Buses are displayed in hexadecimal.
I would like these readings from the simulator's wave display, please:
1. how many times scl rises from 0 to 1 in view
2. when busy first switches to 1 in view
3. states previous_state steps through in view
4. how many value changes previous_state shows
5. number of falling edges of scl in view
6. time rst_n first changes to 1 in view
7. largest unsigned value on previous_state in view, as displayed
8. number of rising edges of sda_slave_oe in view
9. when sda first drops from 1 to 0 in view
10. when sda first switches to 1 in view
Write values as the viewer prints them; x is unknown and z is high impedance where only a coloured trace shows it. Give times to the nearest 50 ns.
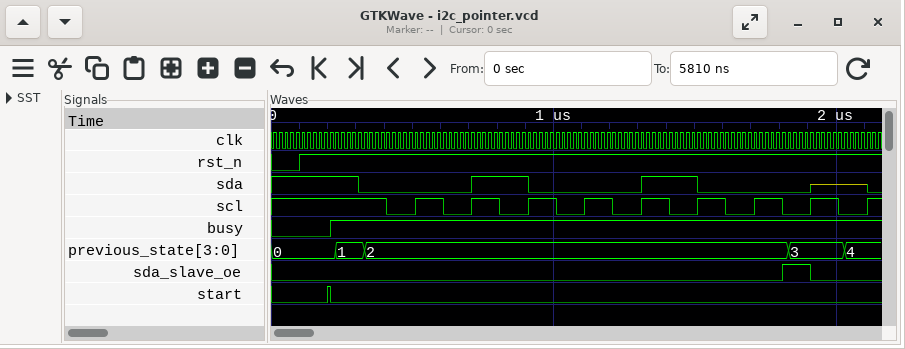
9
200 ns
0, 1, 2, 3, 4
4
9
100 ns
4
1
300 ns
700 ns
